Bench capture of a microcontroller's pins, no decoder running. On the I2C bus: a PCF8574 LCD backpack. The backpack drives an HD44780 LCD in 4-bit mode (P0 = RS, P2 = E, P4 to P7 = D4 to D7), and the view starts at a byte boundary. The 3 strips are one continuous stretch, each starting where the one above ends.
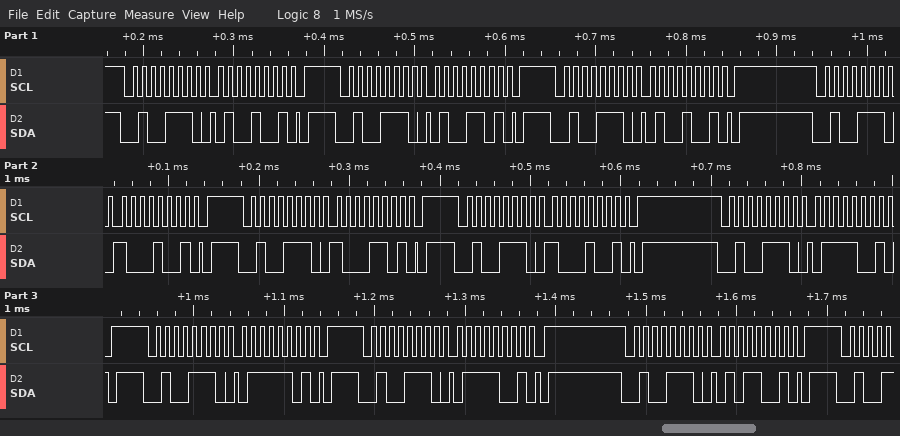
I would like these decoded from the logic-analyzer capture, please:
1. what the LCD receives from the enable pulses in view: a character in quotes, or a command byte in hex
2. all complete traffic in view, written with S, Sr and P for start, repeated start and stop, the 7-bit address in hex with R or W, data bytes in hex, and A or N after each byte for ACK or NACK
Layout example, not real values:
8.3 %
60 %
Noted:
'H'
S 27W A 49 A P S 27W A 4D A P S 27W A 49 A P S 27W A 89 A P S 27W A 8D A P S 27W A 89 A P S 27W A 79 A P S 27W A 7D A P S 27W A 79 A P S 27W A 59 A P
